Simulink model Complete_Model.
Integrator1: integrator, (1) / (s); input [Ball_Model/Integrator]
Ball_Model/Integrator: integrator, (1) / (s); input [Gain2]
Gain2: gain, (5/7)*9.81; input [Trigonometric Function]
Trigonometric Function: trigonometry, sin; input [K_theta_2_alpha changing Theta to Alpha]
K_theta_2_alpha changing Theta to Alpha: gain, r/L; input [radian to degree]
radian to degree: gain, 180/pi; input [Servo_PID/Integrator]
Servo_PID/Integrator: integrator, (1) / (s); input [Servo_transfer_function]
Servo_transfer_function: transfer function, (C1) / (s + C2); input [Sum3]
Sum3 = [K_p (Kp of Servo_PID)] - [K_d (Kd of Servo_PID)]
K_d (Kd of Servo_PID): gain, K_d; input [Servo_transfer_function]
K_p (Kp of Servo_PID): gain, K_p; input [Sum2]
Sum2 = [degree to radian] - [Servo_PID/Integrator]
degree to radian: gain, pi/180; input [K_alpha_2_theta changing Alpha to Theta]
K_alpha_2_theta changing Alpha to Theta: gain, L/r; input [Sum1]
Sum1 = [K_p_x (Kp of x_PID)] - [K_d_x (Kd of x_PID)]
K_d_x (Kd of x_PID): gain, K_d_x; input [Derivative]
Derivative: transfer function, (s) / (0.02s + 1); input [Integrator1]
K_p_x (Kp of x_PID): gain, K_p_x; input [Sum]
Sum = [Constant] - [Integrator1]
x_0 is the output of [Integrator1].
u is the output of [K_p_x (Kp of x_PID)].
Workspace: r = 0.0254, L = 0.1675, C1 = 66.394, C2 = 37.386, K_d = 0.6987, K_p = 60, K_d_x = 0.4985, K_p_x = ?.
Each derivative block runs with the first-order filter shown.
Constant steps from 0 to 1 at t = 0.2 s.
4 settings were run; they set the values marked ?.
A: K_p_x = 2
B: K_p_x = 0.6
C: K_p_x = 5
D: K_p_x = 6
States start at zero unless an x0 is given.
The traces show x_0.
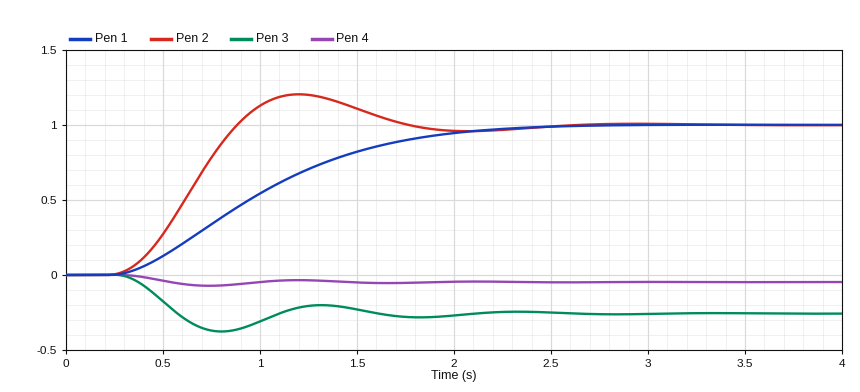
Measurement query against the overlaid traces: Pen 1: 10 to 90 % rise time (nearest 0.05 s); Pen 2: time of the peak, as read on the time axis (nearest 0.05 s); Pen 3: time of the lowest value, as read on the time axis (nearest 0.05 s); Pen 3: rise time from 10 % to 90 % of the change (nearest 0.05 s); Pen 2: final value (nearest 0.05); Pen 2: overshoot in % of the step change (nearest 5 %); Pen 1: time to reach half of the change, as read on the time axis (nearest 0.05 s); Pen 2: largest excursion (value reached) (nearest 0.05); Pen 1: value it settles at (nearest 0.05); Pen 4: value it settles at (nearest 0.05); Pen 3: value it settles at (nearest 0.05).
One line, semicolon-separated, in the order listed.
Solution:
1.30 s; 1.20 s; 0.80 s; 0.20 s; 1.00; 20 %; 0.95 s; 1.20; 1.00; -0.05; -0.25
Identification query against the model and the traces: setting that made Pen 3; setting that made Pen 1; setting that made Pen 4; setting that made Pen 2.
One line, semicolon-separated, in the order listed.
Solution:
C; B; D; A
